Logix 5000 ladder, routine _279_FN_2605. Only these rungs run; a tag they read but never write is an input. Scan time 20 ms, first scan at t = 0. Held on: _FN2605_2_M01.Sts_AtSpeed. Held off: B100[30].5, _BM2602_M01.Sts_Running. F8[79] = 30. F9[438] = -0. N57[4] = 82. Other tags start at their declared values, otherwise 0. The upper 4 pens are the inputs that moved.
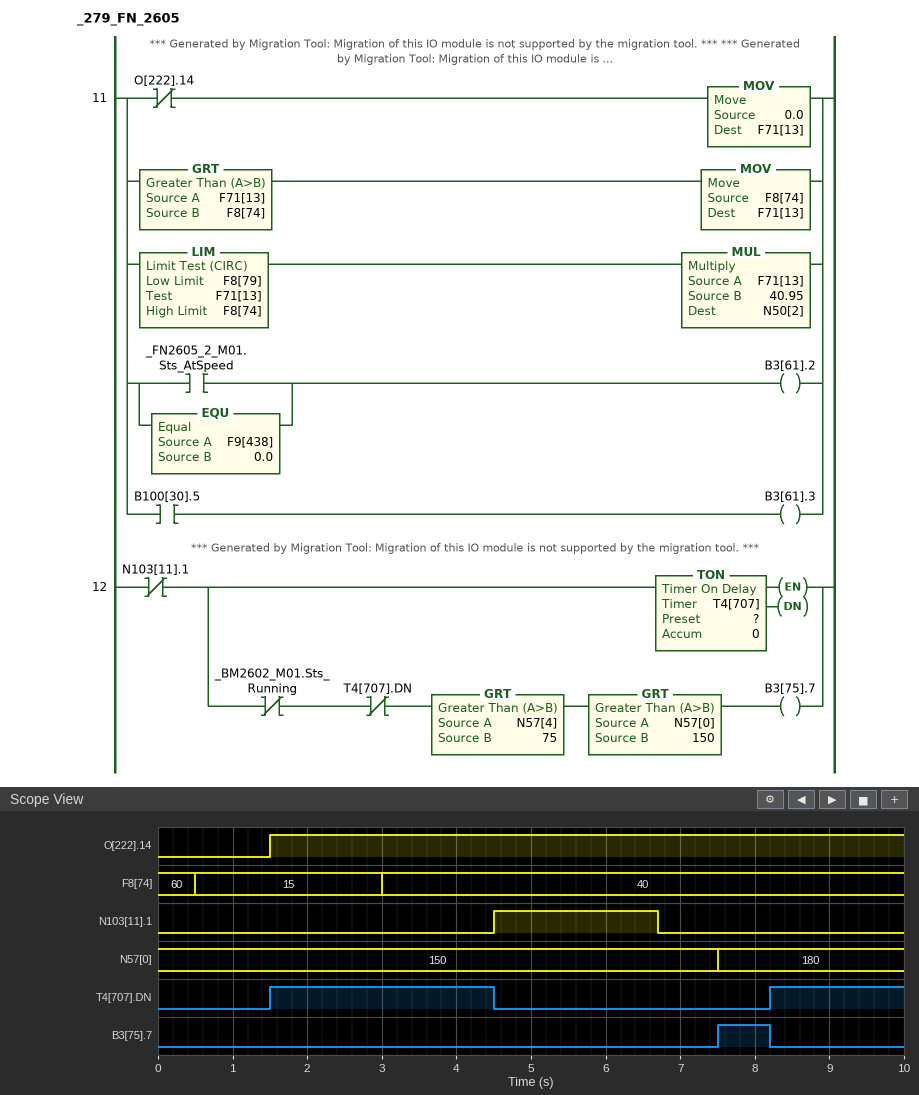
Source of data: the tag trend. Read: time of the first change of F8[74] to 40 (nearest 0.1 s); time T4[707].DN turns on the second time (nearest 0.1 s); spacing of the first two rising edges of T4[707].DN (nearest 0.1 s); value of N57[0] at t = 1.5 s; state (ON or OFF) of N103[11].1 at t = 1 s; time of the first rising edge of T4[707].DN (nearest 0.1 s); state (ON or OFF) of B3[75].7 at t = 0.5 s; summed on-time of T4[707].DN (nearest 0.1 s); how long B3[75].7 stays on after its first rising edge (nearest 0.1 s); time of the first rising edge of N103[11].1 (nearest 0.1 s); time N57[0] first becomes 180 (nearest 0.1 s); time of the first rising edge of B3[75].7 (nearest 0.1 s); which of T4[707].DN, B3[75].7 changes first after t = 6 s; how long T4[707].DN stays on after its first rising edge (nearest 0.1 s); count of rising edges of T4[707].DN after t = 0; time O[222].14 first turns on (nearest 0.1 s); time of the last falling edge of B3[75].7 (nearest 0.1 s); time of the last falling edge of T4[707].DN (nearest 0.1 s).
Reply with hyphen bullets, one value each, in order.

- 3.0 s
- 8.2 s
- 6.7 s
- 150
- OFF
- 1.5 s
- OFF
- 4.8 s
- 0.7 s
- 4.5 s
- 7.5 s
- 7.5 s
- B3[75].7
- 3.0 s
- 2
- 1.5 s
- 8.2 s
- 4.5 s
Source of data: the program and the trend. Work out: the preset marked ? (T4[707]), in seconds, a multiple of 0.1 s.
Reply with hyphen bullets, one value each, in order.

- 1.5 s
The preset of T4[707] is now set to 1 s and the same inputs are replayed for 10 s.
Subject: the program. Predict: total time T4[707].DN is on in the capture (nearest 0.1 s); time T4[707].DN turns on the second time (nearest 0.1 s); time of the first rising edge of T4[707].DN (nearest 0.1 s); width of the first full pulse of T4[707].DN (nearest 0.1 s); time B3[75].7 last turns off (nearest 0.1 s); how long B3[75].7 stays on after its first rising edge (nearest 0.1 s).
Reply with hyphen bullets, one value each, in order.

- 5.8 s
- 7.7 s
- 1.0 s
- 3.5 s
- 7.7 s
- 0.2 s
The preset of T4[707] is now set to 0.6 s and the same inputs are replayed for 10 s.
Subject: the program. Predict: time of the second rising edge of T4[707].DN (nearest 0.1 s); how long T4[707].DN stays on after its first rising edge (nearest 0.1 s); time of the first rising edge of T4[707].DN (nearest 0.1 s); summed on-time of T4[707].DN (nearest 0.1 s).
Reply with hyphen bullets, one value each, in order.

- 7.3 s
- 3.9 s
- 0.6 s
- 6.6 s
